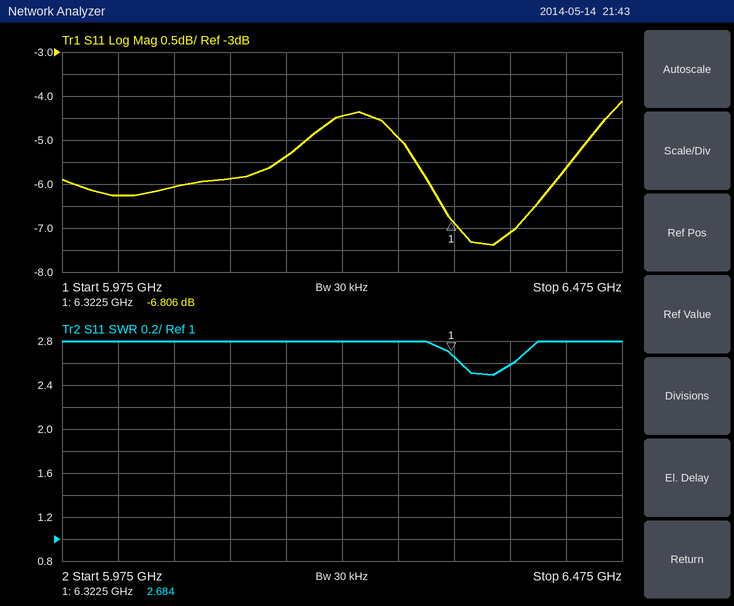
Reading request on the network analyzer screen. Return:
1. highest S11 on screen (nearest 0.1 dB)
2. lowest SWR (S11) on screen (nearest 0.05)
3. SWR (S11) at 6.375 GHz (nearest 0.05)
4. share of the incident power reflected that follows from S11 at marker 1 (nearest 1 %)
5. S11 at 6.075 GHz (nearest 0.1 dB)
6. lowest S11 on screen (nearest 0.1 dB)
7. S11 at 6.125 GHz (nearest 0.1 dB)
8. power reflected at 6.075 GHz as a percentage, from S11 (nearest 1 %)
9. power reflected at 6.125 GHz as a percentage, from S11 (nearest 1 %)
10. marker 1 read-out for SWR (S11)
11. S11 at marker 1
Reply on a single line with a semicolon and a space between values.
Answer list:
-4.1 dB; 2.50; 2.60; 21 %; -6.1 dB; -7.4 dB; -5.9 dB; 25 %; 26 %; 2.684; -6.806 dB
